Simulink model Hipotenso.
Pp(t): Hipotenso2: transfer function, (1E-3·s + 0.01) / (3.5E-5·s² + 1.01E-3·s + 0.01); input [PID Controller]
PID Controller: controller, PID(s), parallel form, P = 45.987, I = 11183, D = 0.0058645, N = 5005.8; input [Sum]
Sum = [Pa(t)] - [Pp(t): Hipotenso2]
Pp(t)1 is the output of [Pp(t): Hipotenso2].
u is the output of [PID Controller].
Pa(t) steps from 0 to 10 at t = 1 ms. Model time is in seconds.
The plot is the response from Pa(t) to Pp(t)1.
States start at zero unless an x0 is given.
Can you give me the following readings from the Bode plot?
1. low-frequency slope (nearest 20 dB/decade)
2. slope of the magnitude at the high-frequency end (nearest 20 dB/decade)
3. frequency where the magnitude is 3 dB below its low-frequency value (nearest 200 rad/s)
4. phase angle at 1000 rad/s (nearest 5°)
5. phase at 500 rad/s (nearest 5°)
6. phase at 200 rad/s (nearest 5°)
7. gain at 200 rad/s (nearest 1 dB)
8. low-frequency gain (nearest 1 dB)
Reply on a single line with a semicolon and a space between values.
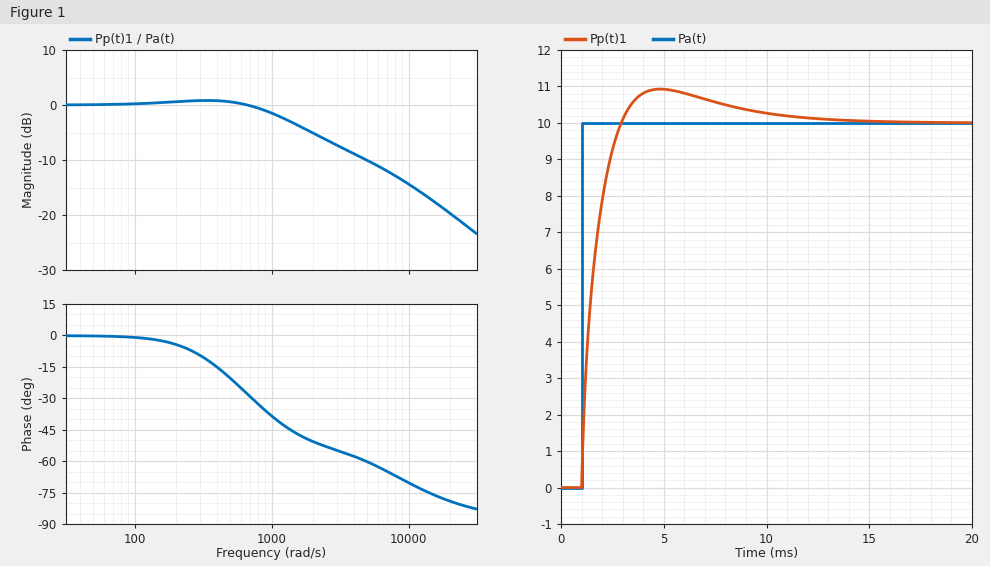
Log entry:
0 dB/decade; -20 dB/decade; 1400 rad/s; -40°; -20°; -5°; 1 dB; 0 dB
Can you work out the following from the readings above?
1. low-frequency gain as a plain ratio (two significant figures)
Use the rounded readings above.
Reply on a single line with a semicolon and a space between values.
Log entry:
1.0
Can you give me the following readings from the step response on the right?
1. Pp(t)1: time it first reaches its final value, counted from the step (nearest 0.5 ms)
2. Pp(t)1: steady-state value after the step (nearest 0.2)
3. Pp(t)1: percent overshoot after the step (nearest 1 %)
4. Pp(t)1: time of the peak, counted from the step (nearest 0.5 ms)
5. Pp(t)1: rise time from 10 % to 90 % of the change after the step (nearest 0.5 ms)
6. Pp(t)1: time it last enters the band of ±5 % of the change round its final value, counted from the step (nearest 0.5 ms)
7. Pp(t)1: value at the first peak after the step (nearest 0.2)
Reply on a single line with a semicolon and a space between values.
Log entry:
2.0 ms; 10.0; 9 %; 4.0 ms; 1.5 ms; 7.0 ms; 11.0
